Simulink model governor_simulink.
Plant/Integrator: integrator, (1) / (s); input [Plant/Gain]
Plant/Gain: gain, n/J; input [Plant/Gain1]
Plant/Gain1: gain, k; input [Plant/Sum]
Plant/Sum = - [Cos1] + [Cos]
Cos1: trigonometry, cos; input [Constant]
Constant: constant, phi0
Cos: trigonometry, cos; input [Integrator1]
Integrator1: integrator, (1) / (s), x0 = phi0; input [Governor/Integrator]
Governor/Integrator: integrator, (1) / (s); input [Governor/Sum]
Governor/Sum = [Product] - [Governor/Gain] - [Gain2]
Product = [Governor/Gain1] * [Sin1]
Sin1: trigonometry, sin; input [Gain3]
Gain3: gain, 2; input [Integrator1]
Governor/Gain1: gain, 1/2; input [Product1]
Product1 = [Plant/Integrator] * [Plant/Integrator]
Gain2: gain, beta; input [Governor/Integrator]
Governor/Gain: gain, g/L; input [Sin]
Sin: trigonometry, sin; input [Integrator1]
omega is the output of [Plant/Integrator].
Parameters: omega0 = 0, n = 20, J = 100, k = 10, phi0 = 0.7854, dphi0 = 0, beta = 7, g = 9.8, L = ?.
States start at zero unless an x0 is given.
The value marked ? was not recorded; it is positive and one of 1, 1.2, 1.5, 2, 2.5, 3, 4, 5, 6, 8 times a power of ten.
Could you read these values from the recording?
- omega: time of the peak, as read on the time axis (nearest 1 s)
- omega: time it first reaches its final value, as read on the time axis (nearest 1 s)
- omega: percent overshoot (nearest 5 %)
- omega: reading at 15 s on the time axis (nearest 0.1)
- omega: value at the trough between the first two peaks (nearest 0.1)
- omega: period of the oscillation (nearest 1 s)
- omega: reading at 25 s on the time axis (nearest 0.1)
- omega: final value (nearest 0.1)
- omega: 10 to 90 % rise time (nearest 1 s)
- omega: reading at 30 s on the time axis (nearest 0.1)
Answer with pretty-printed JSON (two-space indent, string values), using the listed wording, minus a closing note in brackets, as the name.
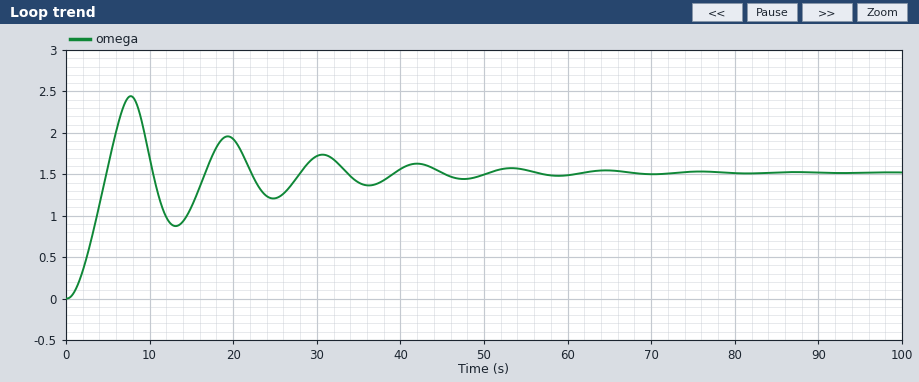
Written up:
{
  "omega: time of the peak, as read on the time axis": "8 s",
  "omega: time it first reaches its final value, as read on the time axis": "5 s",
  "omega: percent overshoot": "60 %",
  "omega: reading at 15 s on the time axis": "1.1",
  "omega: value at the trough between the first two peaks": "0.9",
  "omega: period of the oscillation": "12 s",
  "omega: reading at 25 s on the time axis": "1.2",
  "omega: final value": "1.5",
  "omega: 10 to 90 % rise time": "3 s",
  "omega: reading at 30 s on the time axis": "1.7"
}
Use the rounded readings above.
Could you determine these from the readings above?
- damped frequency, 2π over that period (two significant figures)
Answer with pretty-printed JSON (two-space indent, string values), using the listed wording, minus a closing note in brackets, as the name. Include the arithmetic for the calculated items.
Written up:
{
  "damped frequency, 2π over that period": "2π / 12 = 0.52 rad/s"
}
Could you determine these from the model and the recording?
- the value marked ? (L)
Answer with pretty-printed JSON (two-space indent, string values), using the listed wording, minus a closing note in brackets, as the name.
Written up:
{
  "the value marked ?": "6"
}
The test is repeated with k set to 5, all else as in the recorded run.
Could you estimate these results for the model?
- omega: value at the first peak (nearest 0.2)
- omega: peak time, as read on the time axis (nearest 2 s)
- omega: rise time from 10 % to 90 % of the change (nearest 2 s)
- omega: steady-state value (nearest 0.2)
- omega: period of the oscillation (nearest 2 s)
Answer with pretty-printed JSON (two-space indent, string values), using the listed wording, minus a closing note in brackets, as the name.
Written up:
{
  "omega: value at the first peak": "2.4",
  "omega: peak time, as read on the time axis": "12 s",
  "omega: rise time from 10 % to 90 % of the change": "6 s",
  "omega: steady-state value": "1.6",
  "omega: period of the oscillation": "16 s"
}
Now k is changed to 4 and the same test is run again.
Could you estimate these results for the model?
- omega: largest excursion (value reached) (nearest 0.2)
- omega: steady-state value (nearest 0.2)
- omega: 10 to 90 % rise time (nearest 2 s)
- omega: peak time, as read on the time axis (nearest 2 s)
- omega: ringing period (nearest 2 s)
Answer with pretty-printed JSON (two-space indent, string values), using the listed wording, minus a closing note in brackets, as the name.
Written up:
{
  "omega: largest excursion (value reached)": "2.4",
  "omega: steady-state value": "1.6",
  "omega: 10 to 90 % rise time": "6 s",
  "omega: peak time, as read on the time axis": "14 s",
  "omega: ringing period": "18 s"
}
